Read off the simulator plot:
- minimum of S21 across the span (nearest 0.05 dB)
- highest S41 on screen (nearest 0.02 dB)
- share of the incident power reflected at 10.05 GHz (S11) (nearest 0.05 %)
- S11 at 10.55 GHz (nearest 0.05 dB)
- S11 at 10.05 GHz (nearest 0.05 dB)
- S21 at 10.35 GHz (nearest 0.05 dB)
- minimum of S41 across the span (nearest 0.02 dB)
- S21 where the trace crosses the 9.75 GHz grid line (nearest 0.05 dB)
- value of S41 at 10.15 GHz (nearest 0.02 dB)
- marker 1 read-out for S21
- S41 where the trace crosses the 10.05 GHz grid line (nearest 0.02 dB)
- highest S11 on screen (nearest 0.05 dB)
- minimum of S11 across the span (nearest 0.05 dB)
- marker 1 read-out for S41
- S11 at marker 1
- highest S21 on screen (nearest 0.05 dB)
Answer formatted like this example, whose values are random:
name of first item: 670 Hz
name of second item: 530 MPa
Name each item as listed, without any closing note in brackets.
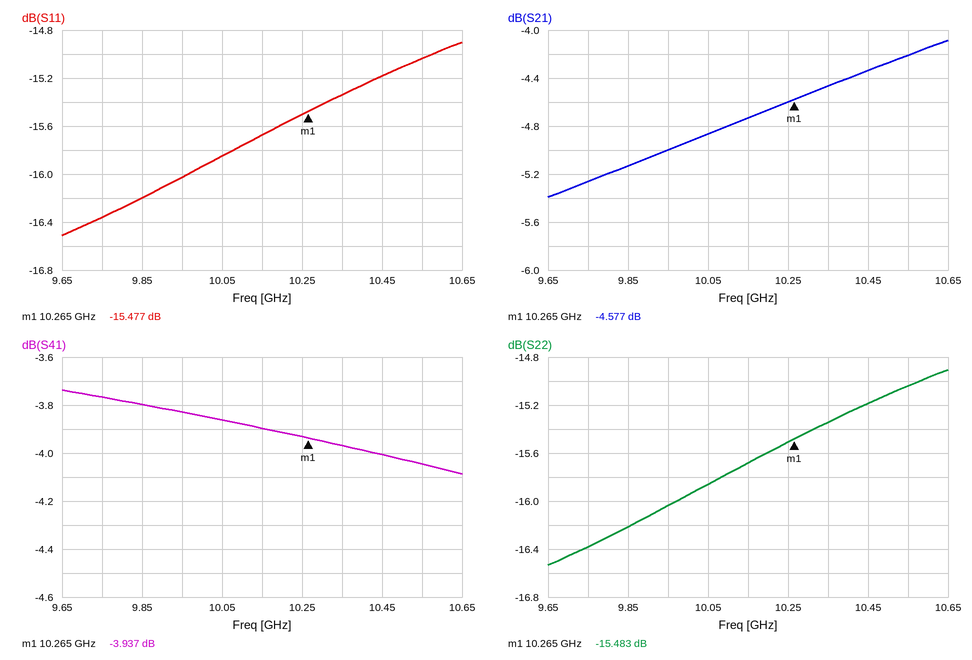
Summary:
minimum of S21 across the span: -5.40 dB
highest S41 on screen: -3.74 dB
share of the incident power reflected at 10.05 GHz (S11): 2.60 %
S11 at 10.55 GHz: -15.05 dB
S11 at 10.05 GHz: -15.85 dB
S21 at 10.35 GHz: -4.45 dB
minimum of S41 across the span: -4.08 dB
S21 where the trace crosses the 9.75 GHz grid line: -5.25 dB
value of S41 at 10.15 GHz: -3.90 dB
marker 1 read-out for S21: -4.577 dB
S41 where the trace crosses the 10.05 GHz grid line: -3.86 dB
highest S11 on screen: -14.90 dB
minimum of S11 across the span: -16.50 dB
marker 1 read-out for S41: -3.937 dB
S11 at marker 1: -15.477 dB
highest S21 on screen: -4.10 dB
